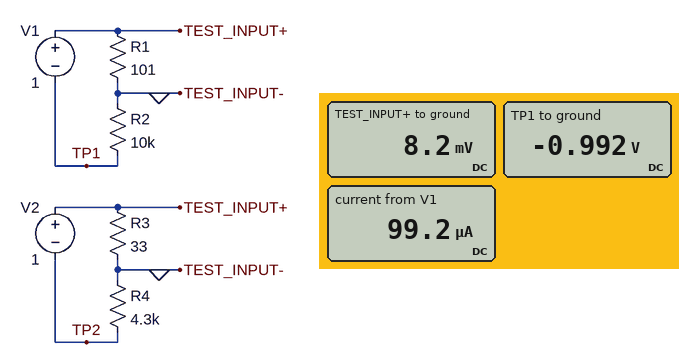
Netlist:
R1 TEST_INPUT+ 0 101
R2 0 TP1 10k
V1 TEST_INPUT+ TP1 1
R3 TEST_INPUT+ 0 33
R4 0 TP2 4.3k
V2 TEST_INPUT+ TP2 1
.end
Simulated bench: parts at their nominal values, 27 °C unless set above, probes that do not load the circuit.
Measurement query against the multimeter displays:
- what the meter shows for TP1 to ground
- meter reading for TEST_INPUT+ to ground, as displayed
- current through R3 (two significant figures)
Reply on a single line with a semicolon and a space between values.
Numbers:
-0.992 V; 8.2 mV; 250 µA
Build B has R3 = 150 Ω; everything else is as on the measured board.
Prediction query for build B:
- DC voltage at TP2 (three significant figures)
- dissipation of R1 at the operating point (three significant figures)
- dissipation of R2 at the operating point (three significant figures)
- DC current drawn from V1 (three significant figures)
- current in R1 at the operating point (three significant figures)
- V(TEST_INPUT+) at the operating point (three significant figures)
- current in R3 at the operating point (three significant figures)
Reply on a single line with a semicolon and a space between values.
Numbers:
-980 mV; 3.83 µW; 96.1 µW; 98.0 µA; 195 µA; 19.7 mV; 131 µA
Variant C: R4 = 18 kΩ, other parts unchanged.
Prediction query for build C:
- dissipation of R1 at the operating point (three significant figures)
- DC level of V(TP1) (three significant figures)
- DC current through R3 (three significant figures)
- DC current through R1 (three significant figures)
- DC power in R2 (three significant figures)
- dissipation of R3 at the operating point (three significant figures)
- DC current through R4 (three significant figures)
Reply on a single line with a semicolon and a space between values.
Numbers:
147 nW; -996 mV; 117 µA; 38.2 µA; 99.2 µW; 450 nW; 55.3 µA
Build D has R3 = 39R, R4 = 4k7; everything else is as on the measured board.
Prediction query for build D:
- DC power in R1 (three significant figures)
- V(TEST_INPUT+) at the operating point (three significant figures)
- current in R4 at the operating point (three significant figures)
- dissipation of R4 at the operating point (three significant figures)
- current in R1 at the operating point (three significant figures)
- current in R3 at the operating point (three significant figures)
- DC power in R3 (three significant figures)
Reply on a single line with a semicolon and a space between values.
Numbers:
753 nW; 8.72 mV; 211 µA; 209 µW; 86.4 µA; 224 µA; 1.95 µW
